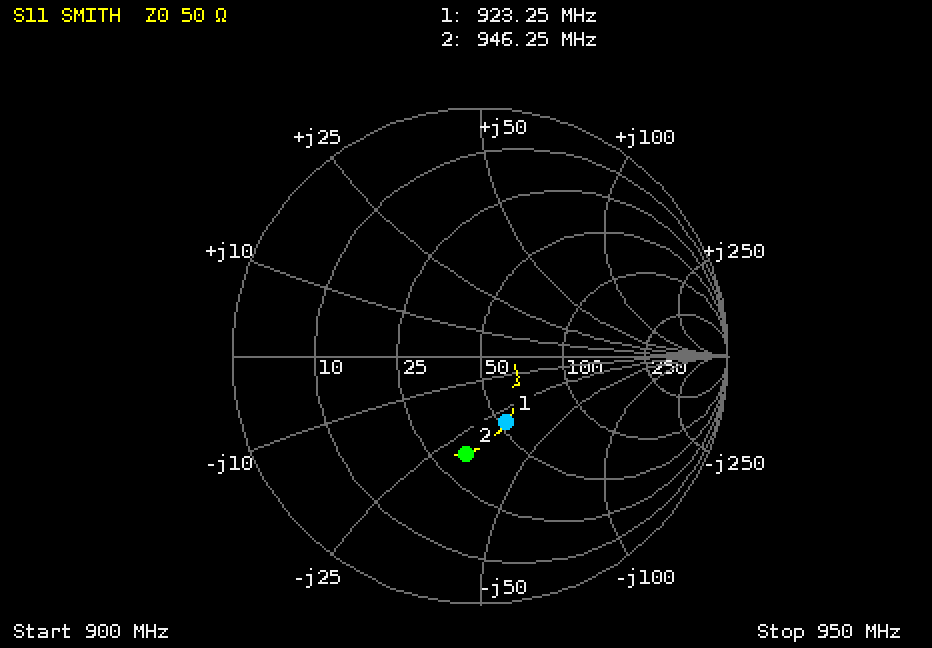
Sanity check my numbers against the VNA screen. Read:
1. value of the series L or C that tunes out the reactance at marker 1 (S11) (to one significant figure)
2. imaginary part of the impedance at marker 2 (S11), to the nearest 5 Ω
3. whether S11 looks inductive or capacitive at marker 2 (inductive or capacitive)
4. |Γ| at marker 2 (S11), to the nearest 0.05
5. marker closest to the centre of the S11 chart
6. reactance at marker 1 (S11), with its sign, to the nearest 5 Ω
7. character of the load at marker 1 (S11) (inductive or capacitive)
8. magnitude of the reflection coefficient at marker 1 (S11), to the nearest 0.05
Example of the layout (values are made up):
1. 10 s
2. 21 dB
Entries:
1. 5 nH
2. -30 Ω
3. capacitive
4. 0.40
5. marker 1
6. -30 Ω
7. capacitive
8. 0.30
